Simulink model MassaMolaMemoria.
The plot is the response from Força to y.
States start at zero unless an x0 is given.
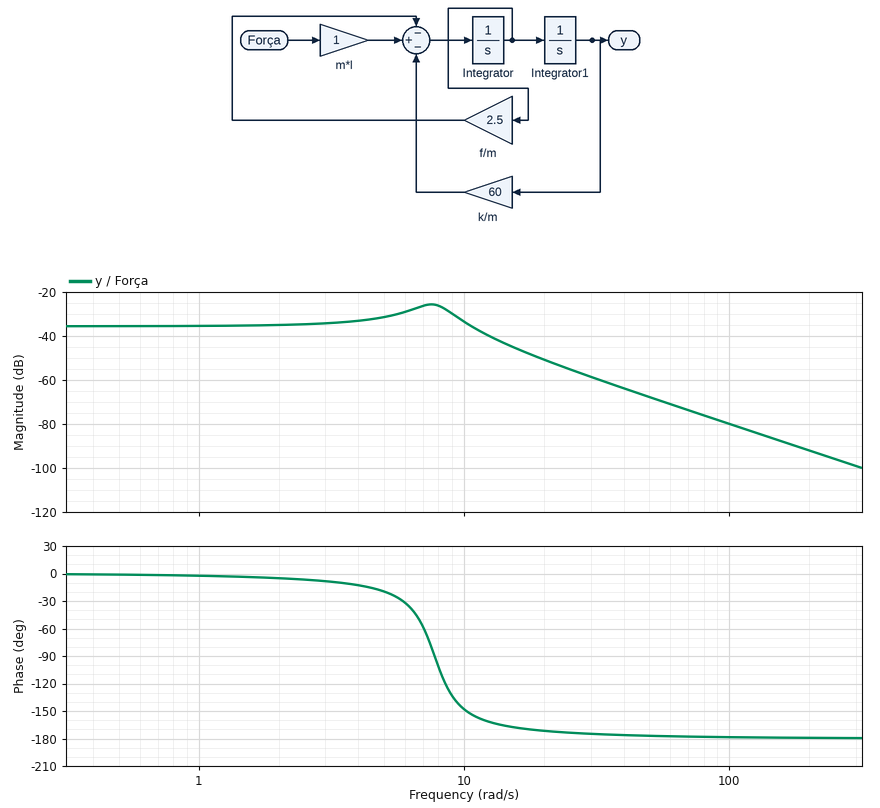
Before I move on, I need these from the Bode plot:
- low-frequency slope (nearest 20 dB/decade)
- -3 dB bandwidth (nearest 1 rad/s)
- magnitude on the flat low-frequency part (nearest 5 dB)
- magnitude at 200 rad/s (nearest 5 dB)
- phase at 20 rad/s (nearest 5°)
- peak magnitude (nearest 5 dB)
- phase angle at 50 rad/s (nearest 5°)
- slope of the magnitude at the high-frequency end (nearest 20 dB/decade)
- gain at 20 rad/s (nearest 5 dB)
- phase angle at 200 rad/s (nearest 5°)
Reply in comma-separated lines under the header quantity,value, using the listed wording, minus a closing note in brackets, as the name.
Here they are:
quantity,value
low-frequency slope,0 dB/decade
-3 dB bandwidth,12 rad/s
magnitude on the flat low-frequency part,-35 dB
magnitude at 200 rad/s,-90 dB
phase at 20 rad/s,-170°
peak magnitude,-25 dB
phase angle at 50 rad/s,-175°
slope of the magnitude at the high-frequency end,-40 dB/decade
gain at 20 rad/s,-50 dB
phase angle at 200 rad/s,-180°
